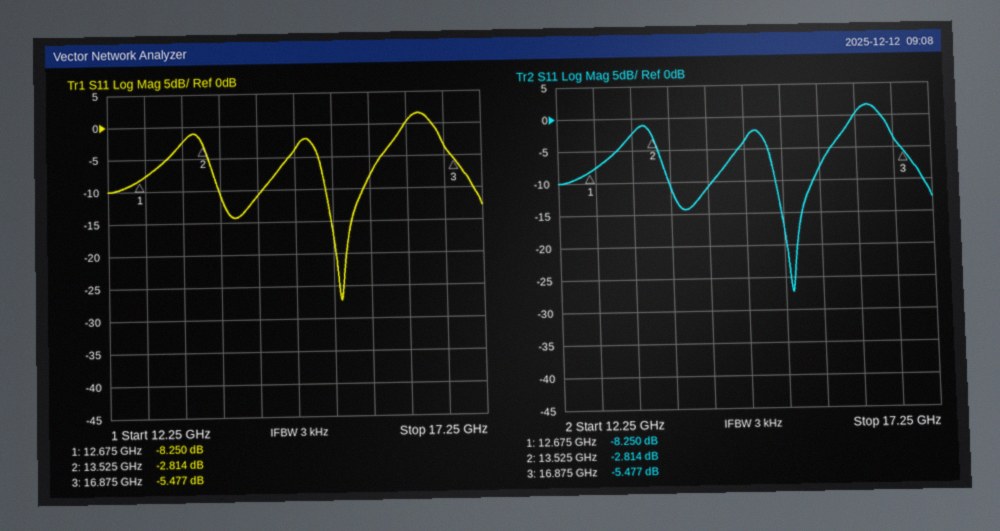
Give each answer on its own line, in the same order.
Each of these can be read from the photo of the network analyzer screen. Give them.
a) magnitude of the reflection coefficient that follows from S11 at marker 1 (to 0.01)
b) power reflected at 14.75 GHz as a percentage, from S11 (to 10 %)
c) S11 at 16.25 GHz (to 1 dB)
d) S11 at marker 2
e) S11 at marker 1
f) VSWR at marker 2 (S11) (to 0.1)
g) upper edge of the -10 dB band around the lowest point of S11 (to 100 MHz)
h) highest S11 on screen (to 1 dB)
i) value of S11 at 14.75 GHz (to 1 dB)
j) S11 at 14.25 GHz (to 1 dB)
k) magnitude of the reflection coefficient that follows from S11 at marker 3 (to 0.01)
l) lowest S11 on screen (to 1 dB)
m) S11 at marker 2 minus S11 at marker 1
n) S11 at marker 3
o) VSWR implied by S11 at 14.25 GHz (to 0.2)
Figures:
0.39
40 %
0 dB
-2.814 dB
-8.250 dB
6.2
15.7 GHz
2 dB
-4 dB
-11 dB
0.53
-27 dB
5.436 dB
-5.477 dB
1.8
